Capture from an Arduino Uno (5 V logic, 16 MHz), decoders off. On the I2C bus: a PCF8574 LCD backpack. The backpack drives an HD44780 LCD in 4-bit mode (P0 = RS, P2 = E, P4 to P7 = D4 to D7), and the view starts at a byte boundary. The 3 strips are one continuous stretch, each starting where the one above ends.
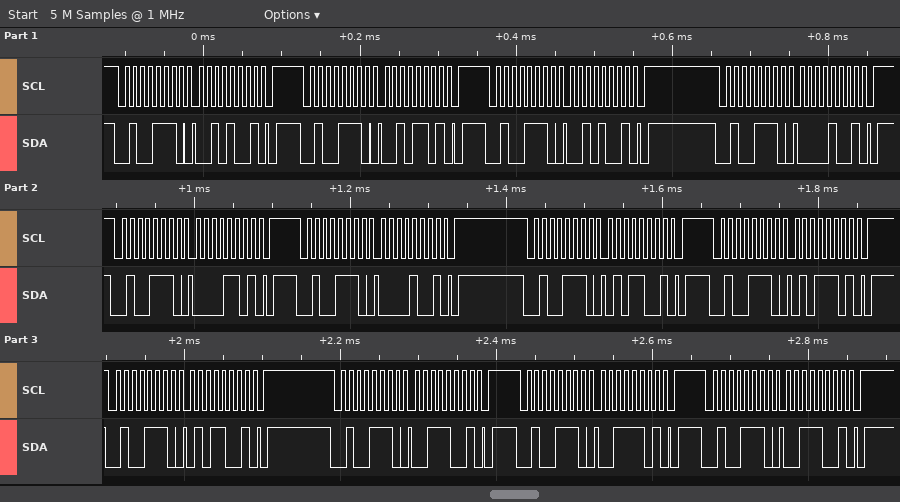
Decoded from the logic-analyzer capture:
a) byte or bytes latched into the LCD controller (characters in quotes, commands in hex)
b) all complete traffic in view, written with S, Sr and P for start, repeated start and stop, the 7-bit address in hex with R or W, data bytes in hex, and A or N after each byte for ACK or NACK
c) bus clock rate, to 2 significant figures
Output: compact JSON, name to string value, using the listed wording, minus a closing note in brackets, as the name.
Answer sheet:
{"byte or bytes latched into the LCD controller": "' ' 'S'", "all complete traffic in view, written with S, Sr and P for start, repeated start and stop, the 7-bit address in hex with R or W, data bytes in hex, and A or N after each byte for ACK or NACK": "S 27W A 29 A P S 27W A 2D A P S 27W A 29 A P S 27W A 09 A P S 27W A 0D A P S 27W A 09 A P S 27W A 59 A P S 27W A 5D A P S 27W A 59 A P S 27W A 39 A P S 27W A 3D A P S 27W A 39 A P", "bus clock rate, to 2 significant figures": "100 kHz"}
